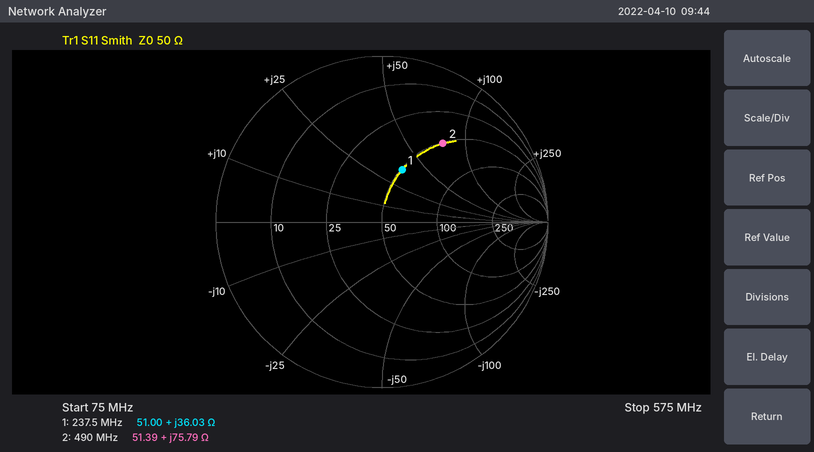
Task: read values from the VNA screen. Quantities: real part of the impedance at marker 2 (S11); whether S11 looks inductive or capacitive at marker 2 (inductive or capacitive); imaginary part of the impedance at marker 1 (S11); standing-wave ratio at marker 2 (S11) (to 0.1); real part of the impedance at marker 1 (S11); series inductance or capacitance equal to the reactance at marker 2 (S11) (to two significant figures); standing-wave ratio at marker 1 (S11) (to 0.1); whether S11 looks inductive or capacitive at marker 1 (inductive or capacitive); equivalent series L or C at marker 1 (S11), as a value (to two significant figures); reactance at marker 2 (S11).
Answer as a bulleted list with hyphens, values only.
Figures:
- 51.39 Ω
- inductive
- +36.03 Ω
- 4.0
- 51.00 Ω
- 25 nH
- 2.0
- inductive
- 24 nH
- +75.79 Ω
